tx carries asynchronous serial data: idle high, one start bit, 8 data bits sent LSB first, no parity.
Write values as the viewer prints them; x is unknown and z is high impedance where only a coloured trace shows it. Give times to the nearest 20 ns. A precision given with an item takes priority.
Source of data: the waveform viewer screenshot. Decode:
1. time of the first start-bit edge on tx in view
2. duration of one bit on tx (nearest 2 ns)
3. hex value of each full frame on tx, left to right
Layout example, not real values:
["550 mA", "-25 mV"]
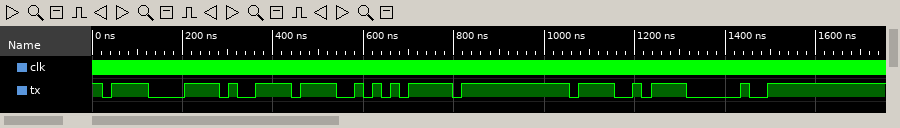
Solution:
["20 ns", "20 ns", "0F, 79, AA, FF, 4F, 20"]
